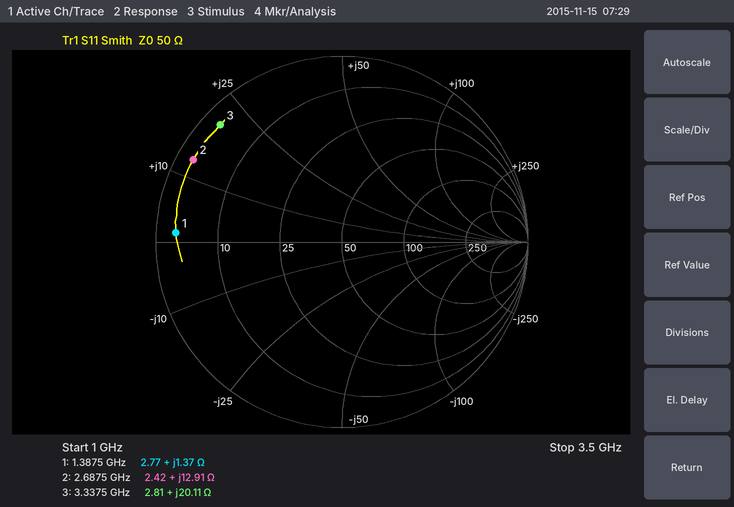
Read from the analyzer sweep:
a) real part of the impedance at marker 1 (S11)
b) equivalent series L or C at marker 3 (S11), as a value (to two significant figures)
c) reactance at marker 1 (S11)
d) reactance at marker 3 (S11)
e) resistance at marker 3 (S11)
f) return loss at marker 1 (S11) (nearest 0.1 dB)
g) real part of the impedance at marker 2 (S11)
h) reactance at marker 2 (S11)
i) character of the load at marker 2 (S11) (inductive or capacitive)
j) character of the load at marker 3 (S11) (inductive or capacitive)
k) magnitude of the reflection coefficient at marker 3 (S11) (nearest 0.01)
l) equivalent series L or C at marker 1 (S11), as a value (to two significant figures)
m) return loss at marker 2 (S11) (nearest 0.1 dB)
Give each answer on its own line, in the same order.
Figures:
2.77 Ω
960 pH
+1.37 Ω
+20.11 Ω
2.81 Ω
1.0 dB
2.42 Ω
+12.91 Ω
inductive
inductive
0.91
160 pH
0.8 dB
